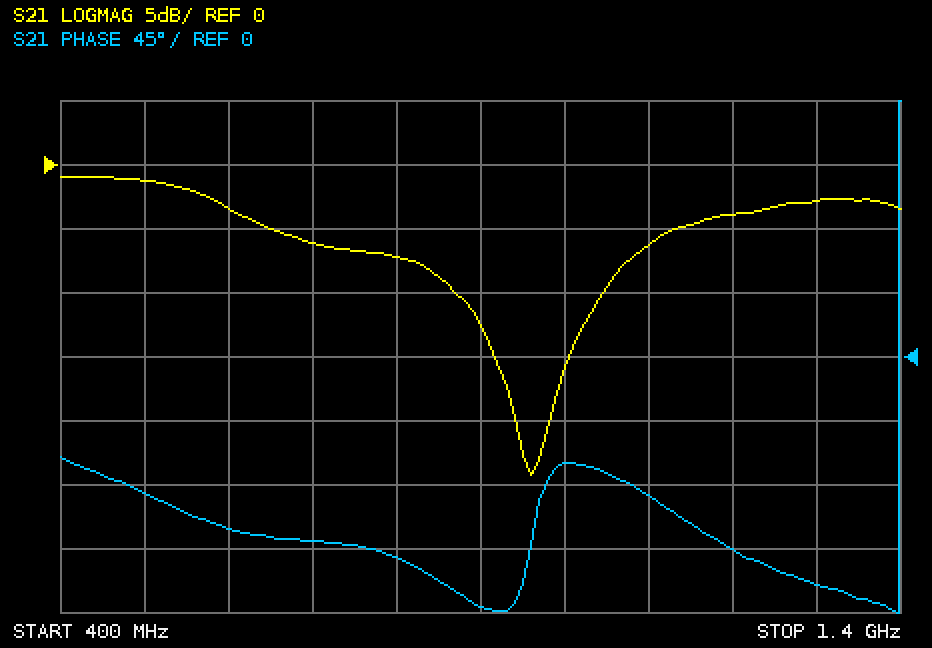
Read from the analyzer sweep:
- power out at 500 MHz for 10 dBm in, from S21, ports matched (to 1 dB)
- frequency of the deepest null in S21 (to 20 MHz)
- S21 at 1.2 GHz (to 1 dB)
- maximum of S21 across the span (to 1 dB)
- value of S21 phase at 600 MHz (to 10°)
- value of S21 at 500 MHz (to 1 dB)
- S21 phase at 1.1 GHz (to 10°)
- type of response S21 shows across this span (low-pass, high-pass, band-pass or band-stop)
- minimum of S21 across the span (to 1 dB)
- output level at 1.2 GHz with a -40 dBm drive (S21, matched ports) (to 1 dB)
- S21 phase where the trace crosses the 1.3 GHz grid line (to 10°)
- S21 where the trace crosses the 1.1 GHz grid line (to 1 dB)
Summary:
9 dBm
960 MHz
-4 dB
-1 dB
-120°
-1 dB
-100°
band-stop
-24 dB
-44 dBm
-160°
-6 dB
